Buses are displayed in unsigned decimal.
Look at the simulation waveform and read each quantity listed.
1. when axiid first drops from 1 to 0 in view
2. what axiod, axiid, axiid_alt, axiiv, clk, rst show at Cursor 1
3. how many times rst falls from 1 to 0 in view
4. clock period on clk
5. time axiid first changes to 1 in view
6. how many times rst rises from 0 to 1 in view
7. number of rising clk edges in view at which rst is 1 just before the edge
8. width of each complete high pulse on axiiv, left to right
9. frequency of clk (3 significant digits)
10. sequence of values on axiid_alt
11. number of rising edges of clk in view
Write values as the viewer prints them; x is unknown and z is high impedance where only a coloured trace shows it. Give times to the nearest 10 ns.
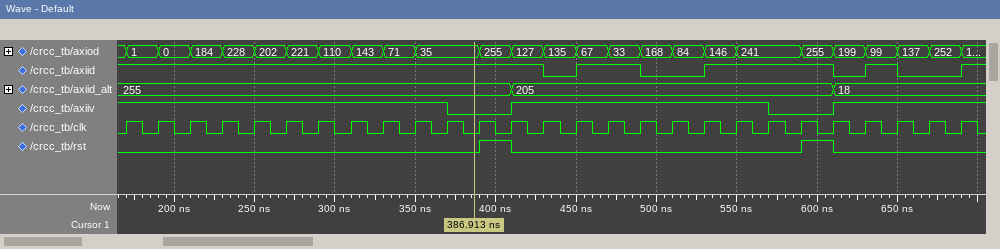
430 ns
axiod=35, axiid=1, axiid_alt=255, axiiv=0, clk=0, rst=0
2
20 ns
450 ns
2
2
160 ns
50.0 MHz
255, 205, 18
27
